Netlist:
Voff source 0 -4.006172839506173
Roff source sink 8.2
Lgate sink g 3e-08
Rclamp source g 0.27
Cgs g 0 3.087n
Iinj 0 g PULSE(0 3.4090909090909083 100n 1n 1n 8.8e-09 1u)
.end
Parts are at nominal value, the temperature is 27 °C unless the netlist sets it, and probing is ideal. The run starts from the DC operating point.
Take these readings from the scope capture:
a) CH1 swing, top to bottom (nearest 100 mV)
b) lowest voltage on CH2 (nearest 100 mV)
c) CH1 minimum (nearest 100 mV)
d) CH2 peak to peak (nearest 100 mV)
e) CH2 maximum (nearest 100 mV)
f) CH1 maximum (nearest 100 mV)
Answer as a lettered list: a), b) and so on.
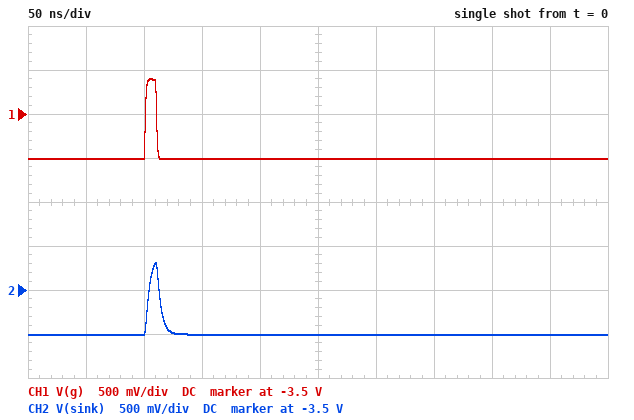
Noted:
a) 900 mV
b) -4.0 V
c) -4.0 V
d) 800 mV
e) -3.2 V
f) -3.1 V
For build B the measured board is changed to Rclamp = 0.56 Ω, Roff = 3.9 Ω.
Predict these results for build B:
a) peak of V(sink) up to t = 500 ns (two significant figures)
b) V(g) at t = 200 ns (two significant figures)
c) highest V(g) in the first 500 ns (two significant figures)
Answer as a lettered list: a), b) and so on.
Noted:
a) -2.8 V
b) -4.0 V
c) -2.2 V
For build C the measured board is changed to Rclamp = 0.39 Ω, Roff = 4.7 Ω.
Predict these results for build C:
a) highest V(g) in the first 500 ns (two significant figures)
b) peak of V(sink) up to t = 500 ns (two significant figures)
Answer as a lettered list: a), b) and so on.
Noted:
a) -2.7 V
b) -3.1 V
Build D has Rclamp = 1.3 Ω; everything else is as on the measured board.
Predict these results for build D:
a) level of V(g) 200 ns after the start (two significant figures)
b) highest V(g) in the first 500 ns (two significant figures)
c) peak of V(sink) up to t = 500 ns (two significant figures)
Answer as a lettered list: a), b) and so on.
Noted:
a) -4.0 V
b) -300 mV
c) -920 mV
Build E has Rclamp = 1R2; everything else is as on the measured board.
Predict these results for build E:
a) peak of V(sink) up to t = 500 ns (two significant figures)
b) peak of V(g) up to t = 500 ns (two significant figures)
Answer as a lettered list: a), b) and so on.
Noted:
a) -1.1 V
b) -510 mV
